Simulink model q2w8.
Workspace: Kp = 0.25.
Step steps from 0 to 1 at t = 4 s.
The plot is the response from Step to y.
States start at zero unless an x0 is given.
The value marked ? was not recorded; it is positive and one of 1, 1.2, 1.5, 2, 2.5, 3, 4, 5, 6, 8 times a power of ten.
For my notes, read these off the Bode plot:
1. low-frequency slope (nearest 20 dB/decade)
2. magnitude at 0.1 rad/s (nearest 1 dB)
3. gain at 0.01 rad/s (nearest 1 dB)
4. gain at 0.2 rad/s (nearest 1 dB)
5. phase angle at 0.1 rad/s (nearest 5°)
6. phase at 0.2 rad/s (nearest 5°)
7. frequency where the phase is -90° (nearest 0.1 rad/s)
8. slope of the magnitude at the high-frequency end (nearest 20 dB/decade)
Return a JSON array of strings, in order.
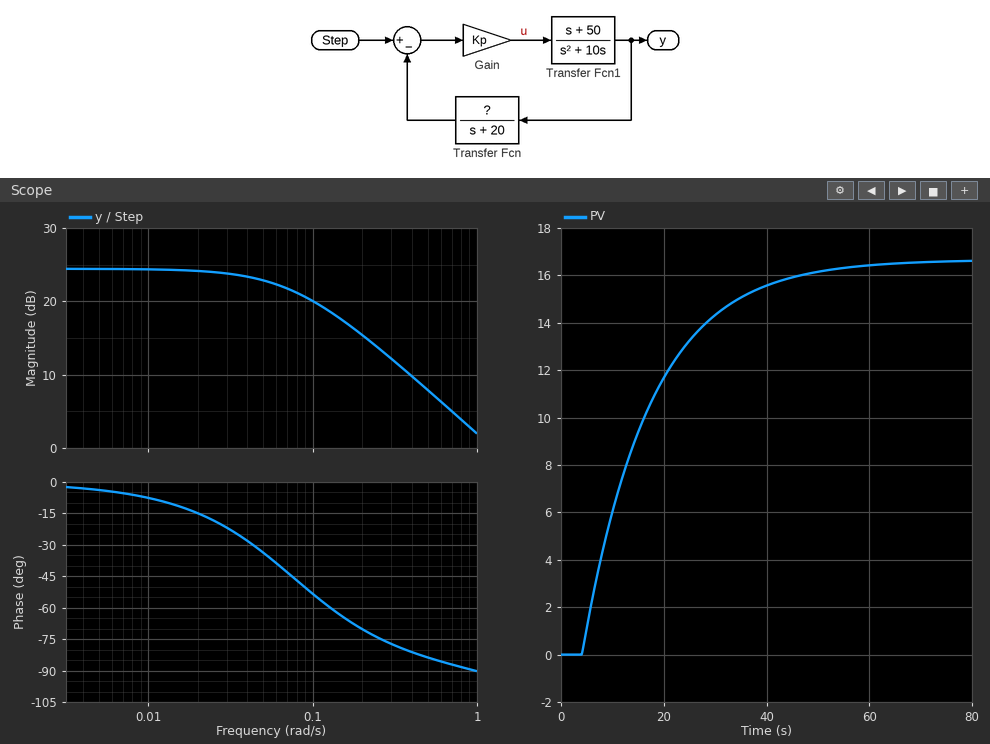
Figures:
["0 dB/decade", "20 dB", "24 dB", "15 dB", "-55°", "-70°", "1.0 rad/s", "-20 dB/decade"]
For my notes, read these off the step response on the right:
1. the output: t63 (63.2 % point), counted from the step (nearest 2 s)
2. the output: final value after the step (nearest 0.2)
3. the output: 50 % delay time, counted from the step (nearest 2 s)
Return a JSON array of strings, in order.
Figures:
["14 s", "16.6", "10 s"]
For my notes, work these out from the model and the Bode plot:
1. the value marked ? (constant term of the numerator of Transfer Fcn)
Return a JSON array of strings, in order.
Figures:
["1.2"]
